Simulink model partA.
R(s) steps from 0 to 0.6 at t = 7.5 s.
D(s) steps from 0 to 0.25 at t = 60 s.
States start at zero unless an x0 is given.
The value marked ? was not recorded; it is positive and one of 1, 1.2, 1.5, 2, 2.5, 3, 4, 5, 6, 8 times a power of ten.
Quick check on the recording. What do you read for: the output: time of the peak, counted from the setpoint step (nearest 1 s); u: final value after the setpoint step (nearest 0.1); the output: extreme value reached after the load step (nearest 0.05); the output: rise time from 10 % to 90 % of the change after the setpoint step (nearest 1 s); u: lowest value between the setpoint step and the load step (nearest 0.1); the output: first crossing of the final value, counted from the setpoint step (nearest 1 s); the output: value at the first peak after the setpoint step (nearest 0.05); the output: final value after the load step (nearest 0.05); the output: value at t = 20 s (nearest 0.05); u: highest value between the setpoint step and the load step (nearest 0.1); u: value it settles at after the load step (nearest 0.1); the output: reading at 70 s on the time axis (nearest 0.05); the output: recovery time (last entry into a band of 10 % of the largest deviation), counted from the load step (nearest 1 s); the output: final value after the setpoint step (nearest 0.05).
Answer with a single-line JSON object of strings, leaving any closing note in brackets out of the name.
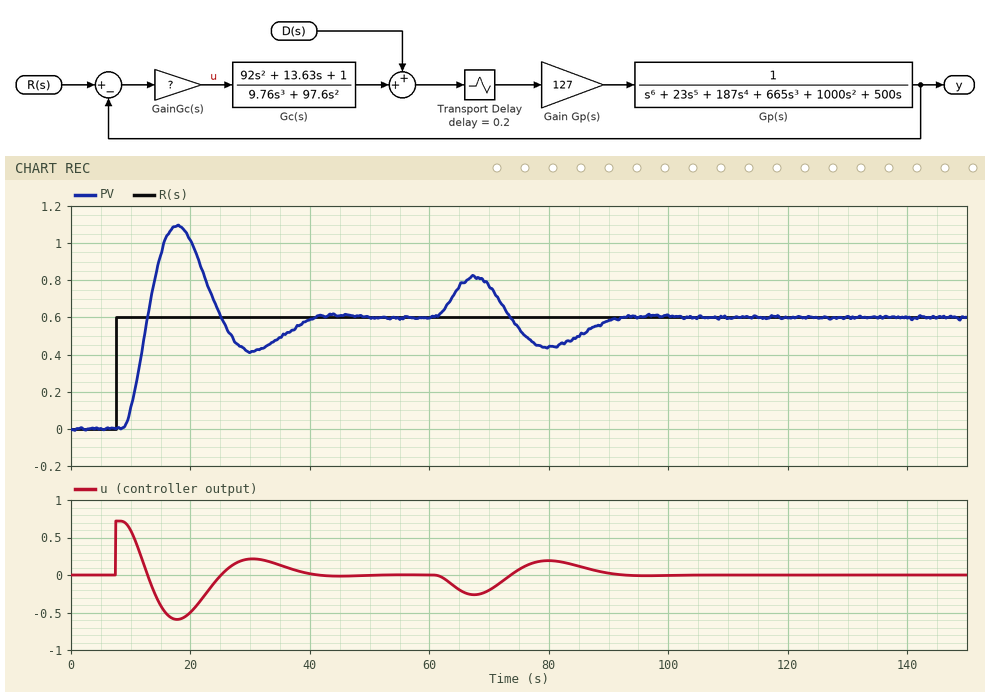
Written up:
{"the output: time of the peak, counted from the setpoint step": "10 s", "u: final value after the setpoint step": "0.0", "the output: extreme value reached after the load step": "0.80", "the output: rise time from 10 % to 90 % of the change after the setpoint step": "3 s", "u: lowest value between the setpoint step and the load step": "-0.6", "the output: first crossing of the final value, counted from the setpoint step": "5 s", "the output: value at the first peak after the setpoint step": "1.10", "the output: final value after the load step": "0.60", "the output: value at t = 20 s": "1.00", "u: highest value between the setpoint step and the load step": "0.7", "u: value it settles at after the load step": "0.0", "the output: reading at 70 s on the time axis": "0.75", "the output: recovery time (last entry into a band of 10 % of the largest deviation), counted from the load step": "30 s", "the output: final value after the setpoint step": "0.60"}
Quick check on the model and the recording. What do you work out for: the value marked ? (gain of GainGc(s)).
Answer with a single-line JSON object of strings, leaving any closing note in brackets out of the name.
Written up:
{"the value marked ? (gain of GainGc(s))": "1.2"}
